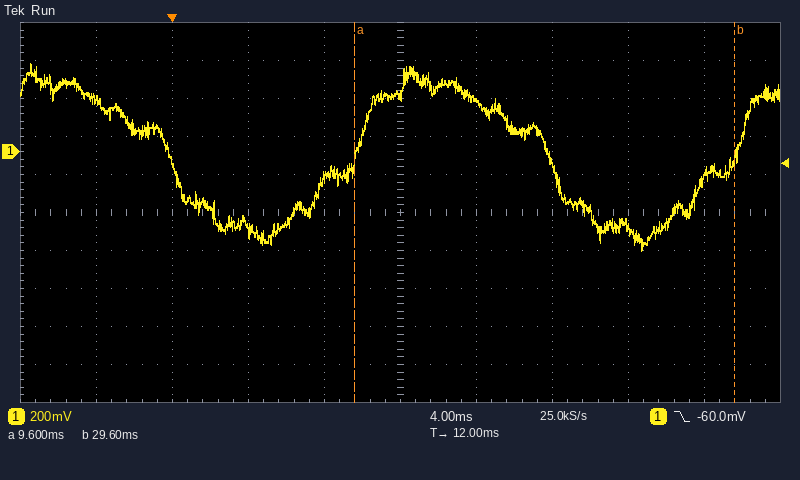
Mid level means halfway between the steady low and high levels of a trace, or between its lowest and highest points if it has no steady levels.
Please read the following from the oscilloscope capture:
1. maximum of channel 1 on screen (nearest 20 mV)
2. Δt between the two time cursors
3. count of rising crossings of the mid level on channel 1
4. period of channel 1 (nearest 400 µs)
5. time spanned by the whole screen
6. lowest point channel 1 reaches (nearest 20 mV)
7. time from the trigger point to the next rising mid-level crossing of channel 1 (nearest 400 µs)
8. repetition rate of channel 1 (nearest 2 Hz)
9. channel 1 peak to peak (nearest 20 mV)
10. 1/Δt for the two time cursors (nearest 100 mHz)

460 mV
20.0 ms
2
20.0 ms
40 ms
-520 mV
9.6 ms
50 Hz
980 mV
50.0 Hz
